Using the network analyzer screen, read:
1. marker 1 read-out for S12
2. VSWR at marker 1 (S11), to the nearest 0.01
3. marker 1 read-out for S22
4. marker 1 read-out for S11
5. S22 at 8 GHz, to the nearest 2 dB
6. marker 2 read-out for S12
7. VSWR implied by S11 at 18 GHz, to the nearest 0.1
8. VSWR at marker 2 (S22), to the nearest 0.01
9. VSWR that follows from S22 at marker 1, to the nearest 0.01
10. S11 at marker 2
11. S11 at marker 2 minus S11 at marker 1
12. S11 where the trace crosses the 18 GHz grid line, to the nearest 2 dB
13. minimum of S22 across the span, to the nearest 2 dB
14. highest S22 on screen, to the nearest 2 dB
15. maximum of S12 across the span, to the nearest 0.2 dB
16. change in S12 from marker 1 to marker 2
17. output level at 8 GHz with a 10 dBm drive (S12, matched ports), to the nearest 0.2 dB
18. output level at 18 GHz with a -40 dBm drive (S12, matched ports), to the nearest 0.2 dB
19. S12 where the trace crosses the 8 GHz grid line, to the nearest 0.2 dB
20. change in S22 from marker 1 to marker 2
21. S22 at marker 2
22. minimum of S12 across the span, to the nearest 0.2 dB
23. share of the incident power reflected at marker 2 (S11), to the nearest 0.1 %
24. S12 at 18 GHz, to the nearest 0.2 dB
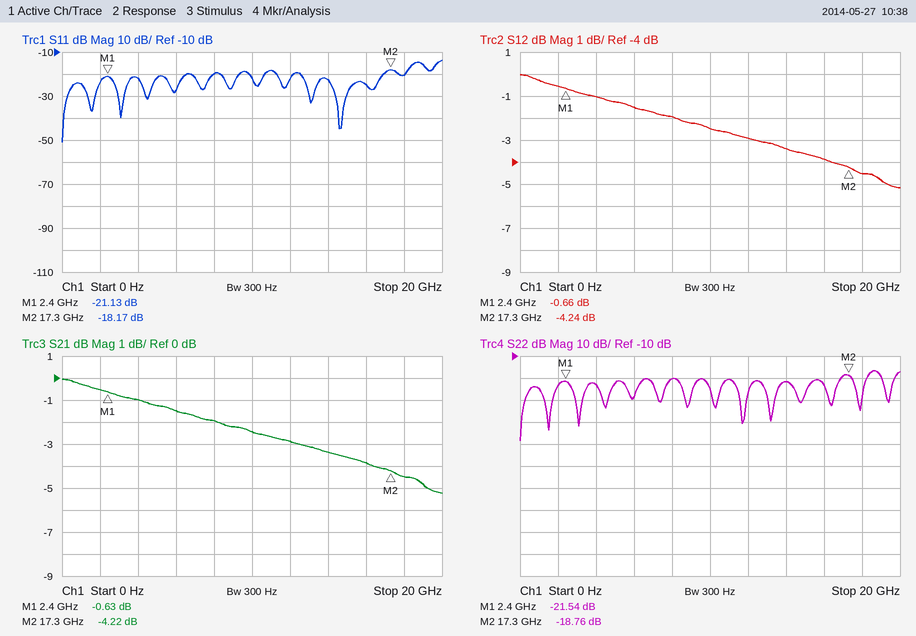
-0.66 dB
1.19
-21.54 dB
-21.13 dB
-20 dB
-4.24 dB
1.2
1.26
1.18
-18.17 dB
2.96 dB
-20 dB
-48 dB
-16 dB
0.0 dB
-3.58 dB
8.0 dBm
-44.6 dBm
-2.0 dB
2.78 dB
-18.76 dB
-5.2 dB
1.5 %
-4.6 dB
